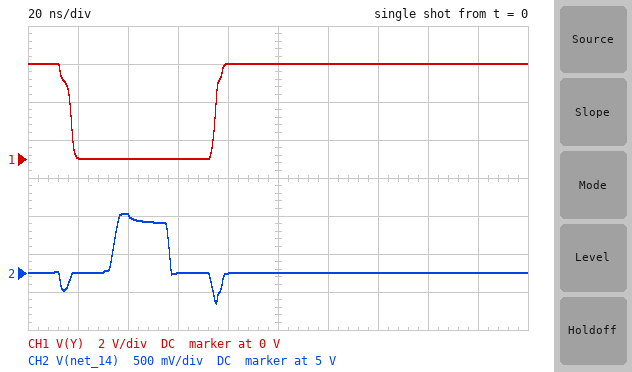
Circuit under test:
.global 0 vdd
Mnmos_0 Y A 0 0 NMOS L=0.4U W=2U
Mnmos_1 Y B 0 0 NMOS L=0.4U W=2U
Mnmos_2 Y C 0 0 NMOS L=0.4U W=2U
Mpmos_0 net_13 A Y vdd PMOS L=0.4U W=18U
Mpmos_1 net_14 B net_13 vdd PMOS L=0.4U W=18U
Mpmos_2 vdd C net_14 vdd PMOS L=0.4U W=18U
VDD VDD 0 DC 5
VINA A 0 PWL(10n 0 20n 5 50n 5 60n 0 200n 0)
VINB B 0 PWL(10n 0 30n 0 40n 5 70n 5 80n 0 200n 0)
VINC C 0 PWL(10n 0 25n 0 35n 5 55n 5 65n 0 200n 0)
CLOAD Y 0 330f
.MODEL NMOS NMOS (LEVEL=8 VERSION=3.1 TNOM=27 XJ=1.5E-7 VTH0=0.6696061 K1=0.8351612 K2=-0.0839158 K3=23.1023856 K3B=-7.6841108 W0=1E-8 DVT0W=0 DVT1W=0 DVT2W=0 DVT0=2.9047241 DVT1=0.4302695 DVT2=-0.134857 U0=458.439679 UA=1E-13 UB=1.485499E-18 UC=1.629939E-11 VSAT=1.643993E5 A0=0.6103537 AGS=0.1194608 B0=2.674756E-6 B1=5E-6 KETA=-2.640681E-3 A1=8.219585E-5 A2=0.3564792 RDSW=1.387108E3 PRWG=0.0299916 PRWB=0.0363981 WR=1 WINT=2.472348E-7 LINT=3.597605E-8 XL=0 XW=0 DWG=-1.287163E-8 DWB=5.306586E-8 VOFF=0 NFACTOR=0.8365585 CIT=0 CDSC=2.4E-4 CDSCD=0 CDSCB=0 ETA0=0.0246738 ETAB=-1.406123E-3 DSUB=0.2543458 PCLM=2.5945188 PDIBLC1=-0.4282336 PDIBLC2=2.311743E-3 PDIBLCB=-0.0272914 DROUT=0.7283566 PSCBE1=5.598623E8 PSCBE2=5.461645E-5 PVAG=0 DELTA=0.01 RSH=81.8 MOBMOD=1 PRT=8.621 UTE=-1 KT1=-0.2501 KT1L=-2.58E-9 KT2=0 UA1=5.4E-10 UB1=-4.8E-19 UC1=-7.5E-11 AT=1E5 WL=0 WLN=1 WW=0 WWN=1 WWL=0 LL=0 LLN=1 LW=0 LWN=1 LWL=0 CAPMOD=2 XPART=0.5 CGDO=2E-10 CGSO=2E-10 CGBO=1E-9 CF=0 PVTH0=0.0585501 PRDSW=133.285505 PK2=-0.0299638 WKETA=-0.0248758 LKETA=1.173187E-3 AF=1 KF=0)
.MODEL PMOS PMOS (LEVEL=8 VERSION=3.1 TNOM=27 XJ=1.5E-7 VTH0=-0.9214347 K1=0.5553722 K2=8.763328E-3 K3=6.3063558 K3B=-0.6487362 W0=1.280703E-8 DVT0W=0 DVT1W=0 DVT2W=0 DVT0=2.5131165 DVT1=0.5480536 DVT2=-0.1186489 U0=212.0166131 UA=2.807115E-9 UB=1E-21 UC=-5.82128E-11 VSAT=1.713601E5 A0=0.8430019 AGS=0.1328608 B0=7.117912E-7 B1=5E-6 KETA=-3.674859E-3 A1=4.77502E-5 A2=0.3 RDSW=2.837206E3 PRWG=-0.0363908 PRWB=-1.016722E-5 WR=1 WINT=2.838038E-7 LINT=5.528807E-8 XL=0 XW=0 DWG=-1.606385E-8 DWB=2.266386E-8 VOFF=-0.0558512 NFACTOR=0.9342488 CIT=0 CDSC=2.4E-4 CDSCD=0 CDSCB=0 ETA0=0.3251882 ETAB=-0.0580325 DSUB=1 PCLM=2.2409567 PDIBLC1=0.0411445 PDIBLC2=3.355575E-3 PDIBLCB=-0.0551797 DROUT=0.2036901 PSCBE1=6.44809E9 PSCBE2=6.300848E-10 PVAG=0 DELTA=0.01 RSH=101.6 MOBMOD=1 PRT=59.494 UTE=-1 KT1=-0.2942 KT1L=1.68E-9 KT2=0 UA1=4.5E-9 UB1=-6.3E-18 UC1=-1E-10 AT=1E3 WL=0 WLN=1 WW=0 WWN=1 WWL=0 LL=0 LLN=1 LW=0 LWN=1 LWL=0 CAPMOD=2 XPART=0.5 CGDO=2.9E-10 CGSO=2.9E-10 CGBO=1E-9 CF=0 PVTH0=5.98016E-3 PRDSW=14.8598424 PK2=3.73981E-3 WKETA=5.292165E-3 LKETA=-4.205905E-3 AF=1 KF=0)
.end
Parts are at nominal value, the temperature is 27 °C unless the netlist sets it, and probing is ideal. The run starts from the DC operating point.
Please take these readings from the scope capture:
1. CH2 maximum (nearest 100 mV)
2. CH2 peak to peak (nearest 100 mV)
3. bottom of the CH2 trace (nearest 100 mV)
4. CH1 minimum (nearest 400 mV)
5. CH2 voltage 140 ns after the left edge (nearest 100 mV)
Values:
5.8 V
1.2 V
4.6 V
0 V
5.0 V
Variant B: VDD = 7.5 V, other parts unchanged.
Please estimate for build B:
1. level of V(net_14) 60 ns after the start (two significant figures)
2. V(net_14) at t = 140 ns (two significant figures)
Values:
7.1 V
7.5 V
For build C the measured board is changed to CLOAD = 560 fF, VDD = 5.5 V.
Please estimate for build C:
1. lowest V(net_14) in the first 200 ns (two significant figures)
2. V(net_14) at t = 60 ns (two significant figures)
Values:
5.0 V
5.5 V
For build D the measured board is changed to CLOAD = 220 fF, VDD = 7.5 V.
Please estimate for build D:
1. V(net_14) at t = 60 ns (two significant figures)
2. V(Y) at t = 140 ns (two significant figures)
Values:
7.1 V
7.5 V
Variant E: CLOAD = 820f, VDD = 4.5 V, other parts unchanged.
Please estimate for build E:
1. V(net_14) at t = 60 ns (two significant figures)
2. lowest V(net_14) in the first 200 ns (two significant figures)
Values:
4.5 V
4.0 V
